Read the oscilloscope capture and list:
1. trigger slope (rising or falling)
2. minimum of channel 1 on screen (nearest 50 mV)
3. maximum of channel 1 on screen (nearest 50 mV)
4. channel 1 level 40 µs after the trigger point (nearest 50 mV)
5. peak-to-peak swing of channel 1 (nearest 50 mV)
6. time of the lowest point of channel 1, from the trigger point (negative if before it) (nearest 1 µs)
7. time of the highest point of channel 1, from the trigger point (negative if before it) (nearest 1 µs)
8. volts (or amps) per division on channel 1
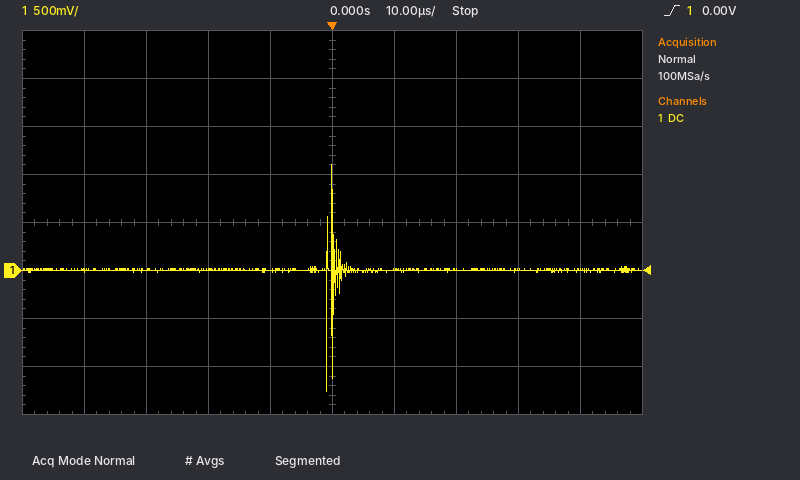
rising
-1.25 V
1.10 V
0 mV
2.35 V
-1 µs
0 µs
500 mV
